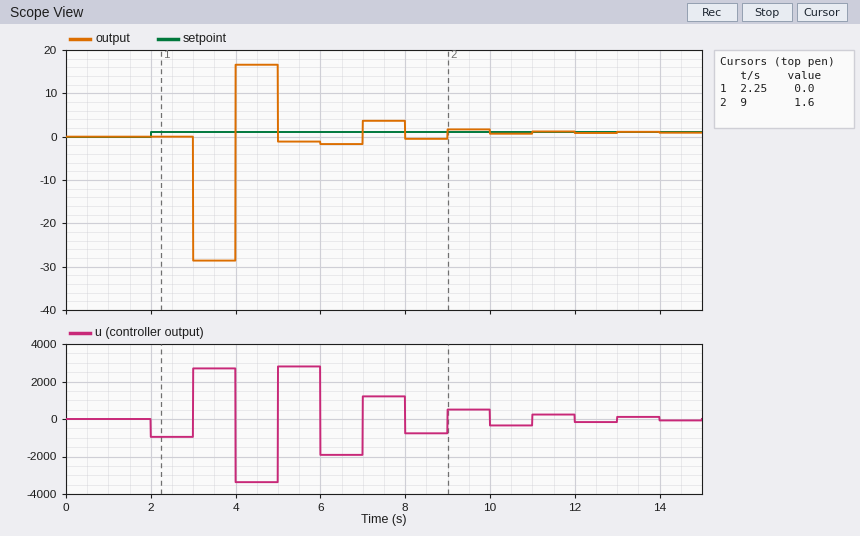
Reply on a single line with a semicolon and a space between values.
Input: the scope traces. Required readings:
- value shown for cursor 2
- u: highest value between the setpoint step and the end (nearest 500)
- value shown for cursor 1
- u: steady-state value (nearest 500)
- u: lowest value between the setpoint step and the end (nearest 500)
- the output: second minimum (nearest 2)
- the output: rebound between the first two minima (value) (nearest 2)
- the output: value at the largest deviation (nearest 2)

1.6; 3000; 0.0; 0; -3500; -2; 16; -28
